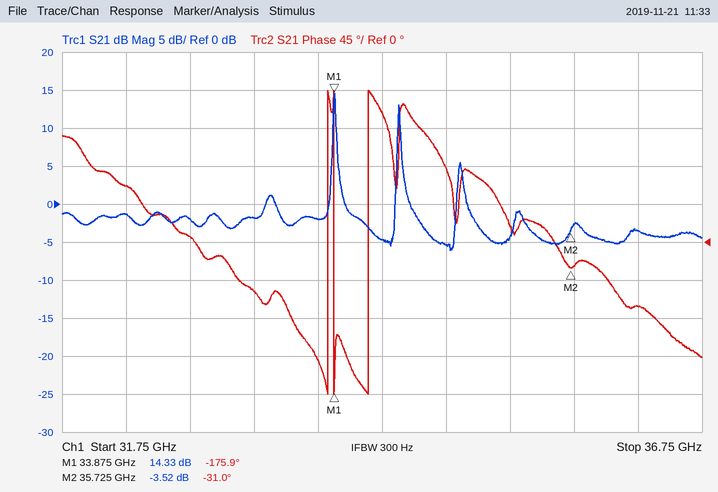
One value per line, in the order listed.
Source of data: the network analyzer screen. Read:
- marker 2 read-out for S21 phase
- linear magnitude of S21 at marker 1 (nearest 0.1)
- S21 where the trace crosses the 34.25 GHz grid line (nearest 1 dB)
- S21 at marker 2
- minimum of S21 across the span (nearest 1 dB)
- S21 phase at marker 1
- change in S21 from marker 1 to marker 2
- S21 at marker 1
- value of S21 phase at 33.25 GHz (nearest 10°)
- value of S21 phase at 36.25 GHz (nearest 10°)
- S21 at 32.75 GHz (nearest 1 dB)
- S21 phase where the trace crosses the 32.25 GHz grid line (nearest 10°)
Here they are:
-31.0°
5.2
-5 dB
-3.52 dB
-6 dB
-175.9°
-17.85 dB
14.33 dB
-60°
-80°
-2 dB
70°
